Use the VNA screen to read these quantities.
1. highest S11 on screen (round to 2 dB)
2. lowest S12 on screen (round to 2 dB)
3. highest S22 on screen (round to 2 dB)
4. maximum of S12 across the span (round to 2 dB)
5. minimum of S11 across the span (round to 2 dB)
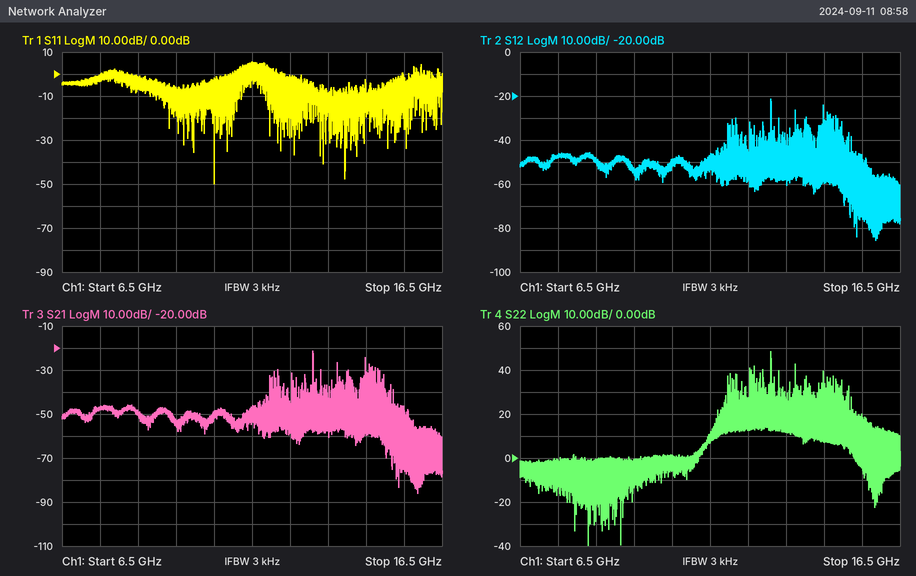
6 dB
-86 dB
48 dB
-22 dB
-50 dB
